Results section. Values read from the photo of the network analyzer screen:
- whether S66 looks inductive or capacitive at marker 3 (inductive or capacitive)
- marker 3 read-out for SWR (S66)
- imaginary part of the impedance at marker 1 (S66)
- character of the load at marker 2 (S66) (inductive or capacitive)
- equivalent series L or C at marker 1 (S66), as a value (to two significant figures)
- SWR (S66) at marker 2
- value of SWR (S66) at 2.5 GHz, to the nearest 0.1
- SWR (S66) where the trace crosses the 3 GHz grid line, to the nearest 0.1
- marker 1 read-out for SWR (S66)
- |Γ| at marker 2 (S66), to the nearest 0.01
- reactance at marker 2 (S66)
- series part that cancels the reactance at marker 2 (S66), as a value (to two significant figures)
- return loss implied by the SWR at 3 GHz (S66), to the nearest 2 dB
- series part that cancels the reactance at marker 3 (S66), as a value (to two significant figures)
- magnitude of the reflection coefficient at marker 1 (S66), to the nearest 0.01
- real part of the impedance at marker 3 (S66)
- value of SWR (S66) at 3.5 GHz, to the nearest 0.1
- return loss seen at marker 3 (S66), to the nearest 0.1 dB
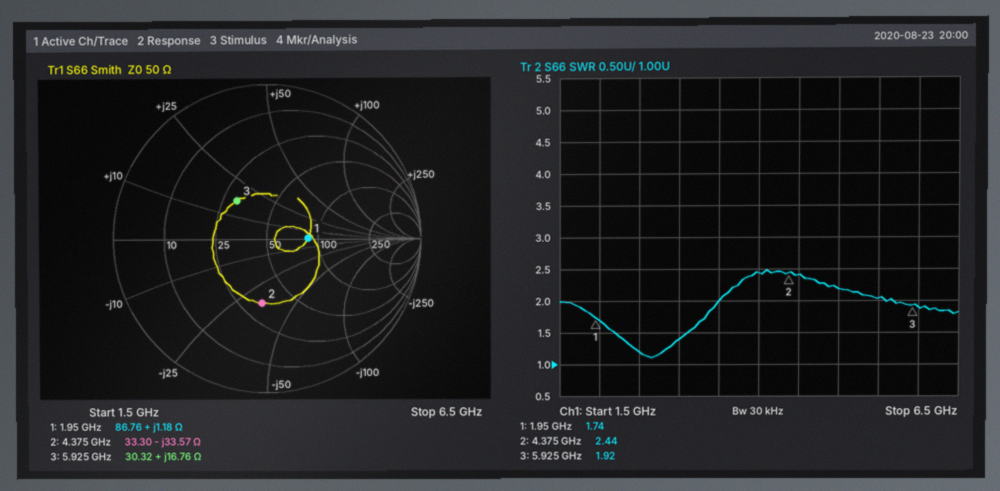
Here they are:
inductive
1.92
+1.18 Ω
capacitive
96 pH
2.44
1.2
1.4
1.74
0.42
-33.57 Ω
1.2 nH
16 dB
1.6 pF
0.27
30.32 Ω
2.0
10.0 dB
